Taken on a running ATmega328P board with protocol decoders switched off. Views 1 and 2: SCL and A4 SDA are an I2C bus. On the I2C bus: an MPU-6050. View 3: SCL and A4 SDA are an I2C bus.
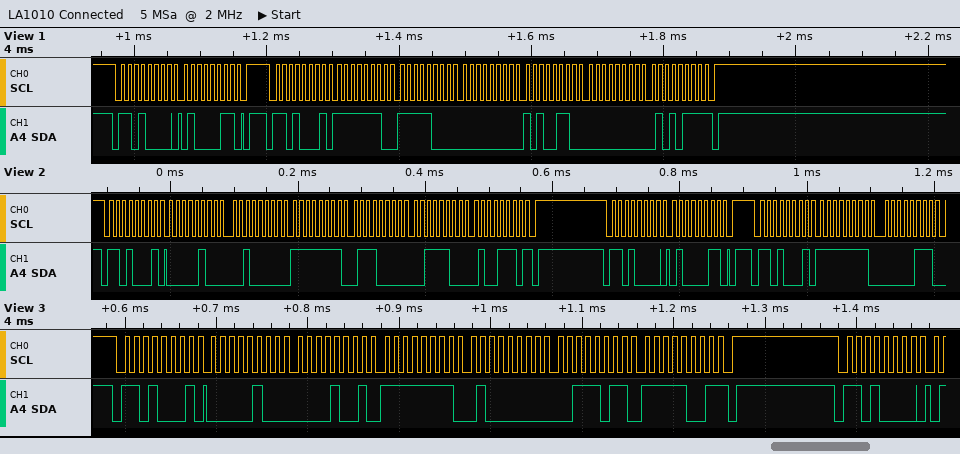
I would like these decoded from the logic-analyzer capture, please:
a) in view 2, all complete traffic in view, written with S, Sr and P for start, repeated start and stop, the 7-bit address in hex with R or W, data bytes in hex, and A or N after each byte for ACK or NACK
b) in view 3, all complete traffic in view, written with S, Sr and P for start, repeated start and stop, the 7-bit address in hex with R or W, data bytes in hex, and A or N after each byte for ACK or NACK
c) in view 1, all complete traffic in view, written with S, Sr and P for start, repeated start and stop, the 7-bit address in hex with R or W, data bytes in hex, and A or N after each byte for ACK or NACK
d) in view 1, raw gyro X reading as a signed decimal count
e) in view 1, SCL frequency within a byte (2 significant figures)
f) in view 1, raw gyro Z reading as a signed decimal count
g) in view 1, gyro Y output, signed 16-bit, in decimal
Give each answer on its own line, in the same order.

S 68R A 04 A 20 A FF A 70 A 3C A 4E N P S 68W A 43 A P S 68R A FF A 07 A
S 68R A 04 A 09 A FF A 40 A 3B A F9 N P S 68W A
S 68W A 43 A P S 68R A FE A F8 A 00 A A6 A 00 A 57 N P
-264
100 kHz
87
166
